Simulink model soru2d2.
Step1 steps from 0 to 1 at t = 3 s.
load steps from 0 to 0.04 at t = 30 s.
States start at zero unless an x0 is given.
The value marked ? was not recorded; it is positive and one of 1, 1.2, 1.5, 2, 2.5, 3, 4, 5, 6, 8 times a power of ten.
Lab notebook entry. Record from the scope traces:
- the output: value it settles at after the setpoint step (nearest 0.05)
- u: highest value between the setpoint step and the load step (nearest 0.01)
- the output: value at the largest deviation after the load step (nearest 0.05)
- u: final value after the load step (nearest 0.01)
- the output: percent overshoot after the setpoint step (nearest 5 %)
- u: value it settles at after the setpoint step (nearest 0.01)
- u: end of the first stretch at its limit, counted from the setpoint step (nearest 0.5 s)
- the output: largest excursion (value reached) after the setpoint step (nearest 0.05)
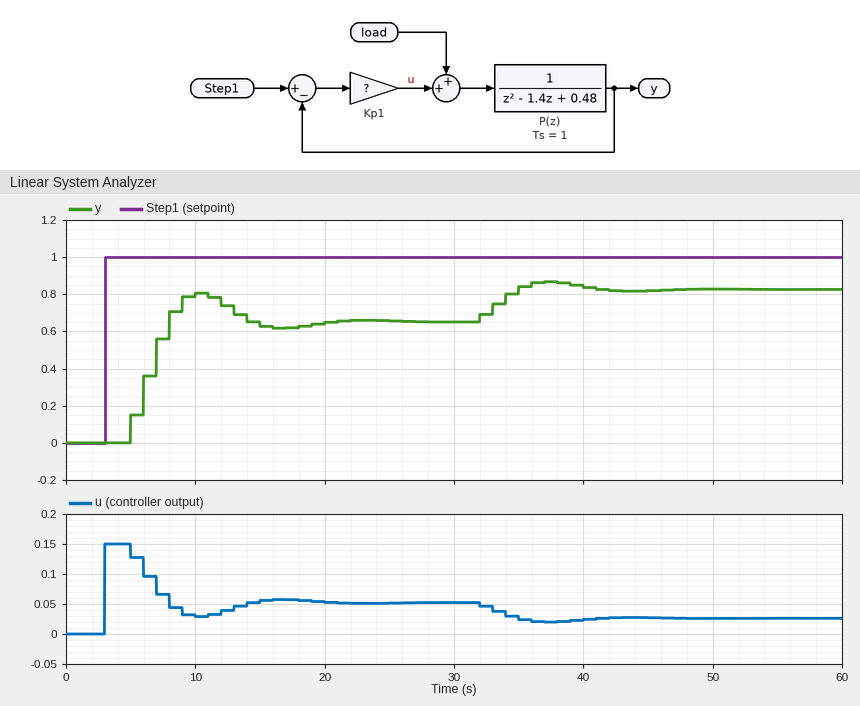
0.65
0.15
0.85
0.03
25 %
0.05
2.0 s
0.80
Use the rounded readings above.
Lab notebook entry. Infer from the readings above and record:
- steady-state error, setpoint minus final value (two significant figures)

0.35
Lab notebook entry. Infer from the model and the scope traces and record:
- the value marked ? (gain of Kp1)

0.15
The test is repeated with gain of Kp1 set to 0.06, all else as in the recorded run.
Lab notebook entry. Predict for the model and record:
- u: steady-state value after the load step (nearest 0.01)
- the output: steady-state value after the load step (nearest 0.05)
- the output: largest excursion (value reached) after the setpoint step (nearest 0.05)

0.02
0.70
0.45
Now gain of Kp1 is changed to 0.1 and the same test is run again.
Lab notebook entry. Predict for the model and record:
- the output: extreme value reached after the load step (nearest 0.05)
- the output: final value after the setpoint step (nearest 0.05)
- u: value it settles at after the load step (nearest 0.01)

0.80
0.55
0.02
